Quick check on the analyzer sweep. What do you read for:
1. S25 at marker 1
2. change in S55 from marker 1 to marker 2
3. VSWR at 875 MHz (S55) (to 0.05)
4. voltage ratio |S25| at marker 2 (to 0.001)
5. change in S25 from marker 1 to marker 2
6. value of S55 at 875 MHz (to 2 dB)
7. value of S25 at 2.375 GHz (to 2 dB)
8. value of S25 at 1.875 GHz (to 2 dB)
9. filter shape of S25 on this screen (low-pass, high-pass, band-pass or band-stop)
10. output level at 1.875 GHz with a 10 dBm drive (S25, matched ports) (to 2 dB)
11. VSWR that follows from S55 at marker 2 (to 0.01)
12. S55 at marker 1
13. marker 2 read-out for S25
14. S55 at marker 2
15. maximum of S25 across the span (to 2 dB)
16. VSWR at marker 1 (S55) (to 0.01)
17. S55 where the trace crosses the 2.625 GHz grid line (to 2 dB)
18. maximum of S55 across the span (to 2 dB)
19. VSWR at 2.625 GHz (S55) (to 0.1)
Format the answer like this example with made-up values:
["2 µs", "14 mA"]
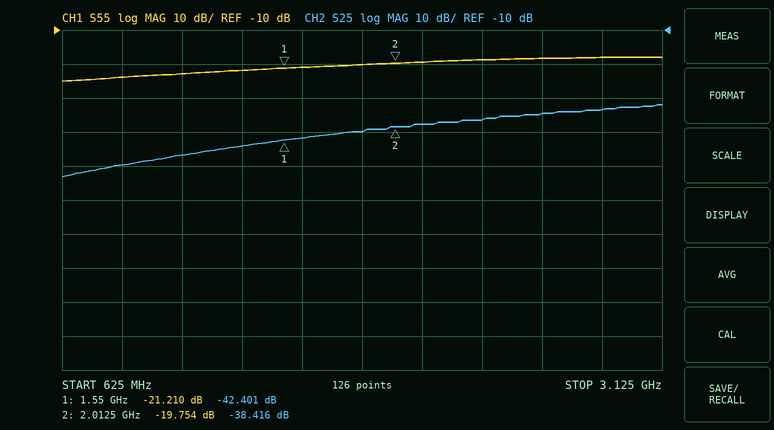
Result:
["-42.401 dB", "1.456 dB", "1.15", "0.012", "3.985 dB", "-24 dB", "-36 dB", "-40 dB", "high-pass", "-30 dBm", "1.23", "-21.210 dB", "-38.416 dB", "-19.754 dB", "-32 dB", "1.19", "-18 dB", "-18 dB", "1.3"]
